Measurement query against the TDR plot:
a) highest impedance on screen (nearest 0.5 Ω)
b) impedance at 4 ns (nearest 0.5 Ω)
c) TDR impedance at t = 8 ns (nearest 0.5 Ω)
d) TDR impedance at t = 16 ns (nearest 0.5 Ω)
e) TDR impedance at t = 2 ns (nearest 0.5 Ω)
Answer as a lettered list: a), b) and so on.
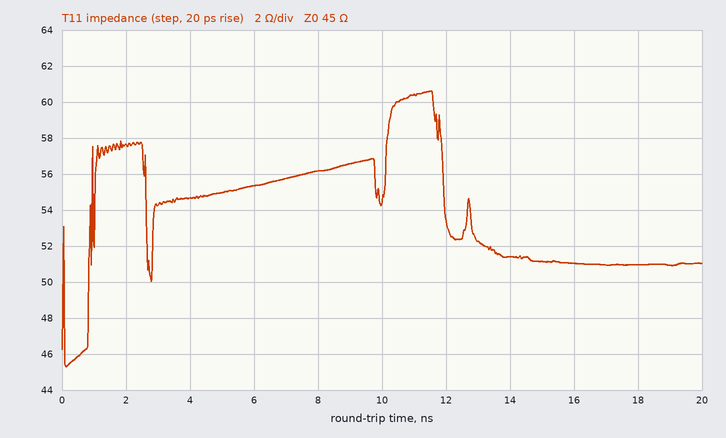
a) 60.5 Ω
b) 54.5 Ω
c) 56.0 Ω
d) 51.0 Ω
e) 57.5 Ω
